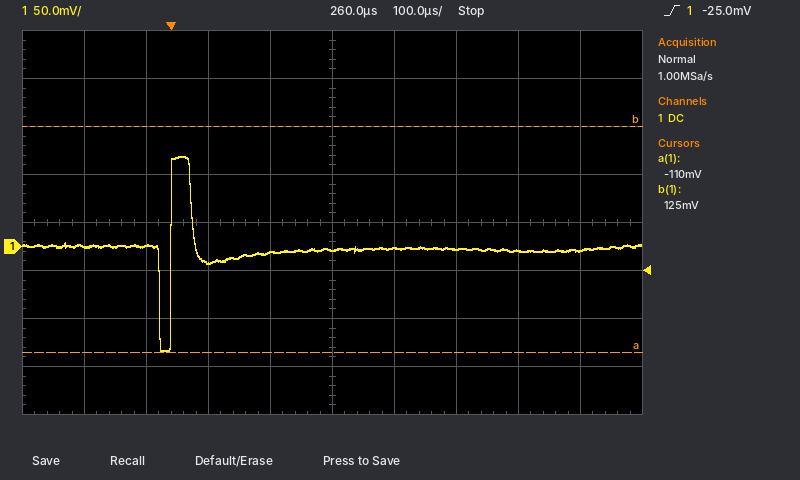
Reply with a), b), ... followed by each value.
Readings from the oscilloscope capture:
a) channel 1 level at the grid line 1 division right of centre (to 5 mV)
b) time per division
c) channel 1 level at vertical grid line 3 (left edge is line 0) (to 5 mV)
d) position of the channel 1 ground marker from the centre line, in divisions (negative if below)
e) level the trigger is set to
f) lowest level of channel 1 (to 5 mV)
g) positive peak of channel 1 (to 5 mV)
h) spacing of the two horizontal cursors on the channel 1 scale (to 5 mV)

a) 0 mV
b) 100 µs
c) -15 mV
d) -0.5 div
e) -25.0 mV
f) -110 mV
g) 95 mV
h) 235 mV
